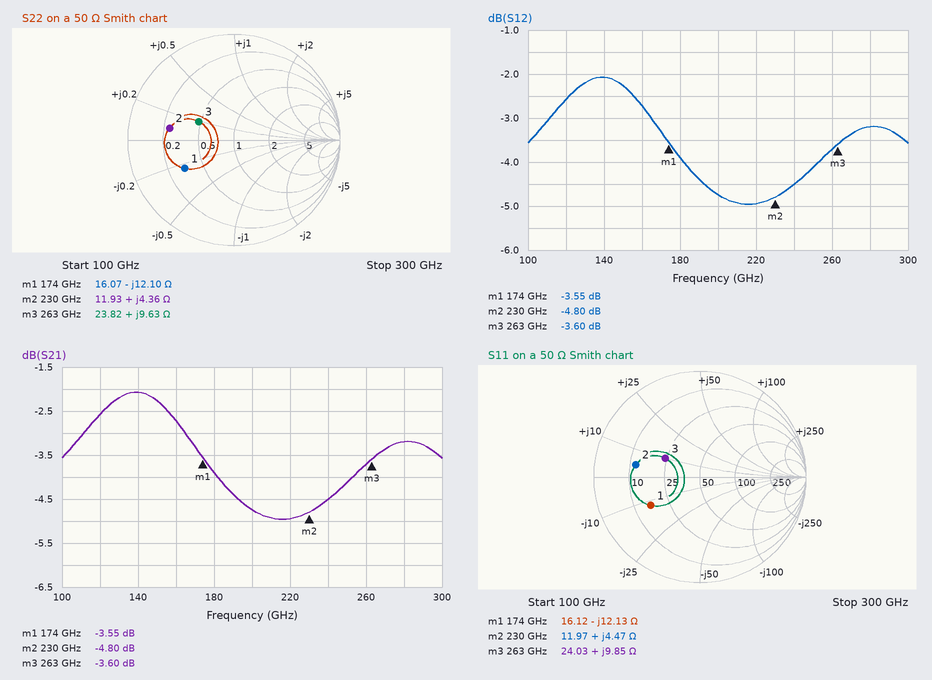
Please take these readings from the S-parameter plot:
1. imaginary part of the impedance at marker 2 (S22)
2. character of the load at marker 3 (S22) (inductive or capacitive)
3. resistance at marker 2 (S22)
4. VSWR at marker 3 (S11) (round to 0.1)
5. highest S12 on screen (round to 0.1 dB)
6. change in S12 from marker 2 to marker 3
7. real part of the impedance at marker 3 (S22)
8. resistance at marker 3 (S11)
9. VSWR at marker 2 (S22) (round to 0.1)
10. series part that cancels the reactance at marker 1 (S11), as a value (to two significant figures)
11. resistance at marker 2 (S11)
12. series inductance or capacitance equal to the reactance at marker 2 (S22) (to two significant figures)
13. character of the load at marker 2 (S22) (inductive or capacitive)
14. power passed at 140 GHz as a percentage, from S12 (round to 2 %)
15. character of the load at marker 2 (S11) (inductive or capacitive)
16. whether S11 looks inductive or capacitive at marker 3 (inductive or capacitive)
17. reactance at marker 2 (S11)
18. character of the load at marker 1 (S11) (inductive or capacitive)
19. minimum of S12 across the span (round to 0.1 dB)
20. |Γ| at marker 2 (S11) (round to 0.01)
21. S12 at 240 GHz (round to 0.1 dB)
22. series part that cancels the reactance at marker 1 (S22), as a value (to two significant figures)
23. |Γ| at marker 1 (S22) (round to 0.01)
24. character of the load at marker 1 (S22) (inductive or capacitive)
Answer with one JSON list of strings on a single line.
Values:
["+4.36 Ω", "inductive", "11.93 Ω", "2.2", "-2.1 dB", "1.20 dB", "23.82 Ω", "24.03 Ω", "4.2", "11 pH", "11.97 Ω", "3.0 pH", "inductive", "62 %", "inductive", "inductive", "+4.47 Ω", "capacitive", "-5.0 dB", "0.62", "-4.5 dB", "11 pH", "0.54", "capacitive"]
